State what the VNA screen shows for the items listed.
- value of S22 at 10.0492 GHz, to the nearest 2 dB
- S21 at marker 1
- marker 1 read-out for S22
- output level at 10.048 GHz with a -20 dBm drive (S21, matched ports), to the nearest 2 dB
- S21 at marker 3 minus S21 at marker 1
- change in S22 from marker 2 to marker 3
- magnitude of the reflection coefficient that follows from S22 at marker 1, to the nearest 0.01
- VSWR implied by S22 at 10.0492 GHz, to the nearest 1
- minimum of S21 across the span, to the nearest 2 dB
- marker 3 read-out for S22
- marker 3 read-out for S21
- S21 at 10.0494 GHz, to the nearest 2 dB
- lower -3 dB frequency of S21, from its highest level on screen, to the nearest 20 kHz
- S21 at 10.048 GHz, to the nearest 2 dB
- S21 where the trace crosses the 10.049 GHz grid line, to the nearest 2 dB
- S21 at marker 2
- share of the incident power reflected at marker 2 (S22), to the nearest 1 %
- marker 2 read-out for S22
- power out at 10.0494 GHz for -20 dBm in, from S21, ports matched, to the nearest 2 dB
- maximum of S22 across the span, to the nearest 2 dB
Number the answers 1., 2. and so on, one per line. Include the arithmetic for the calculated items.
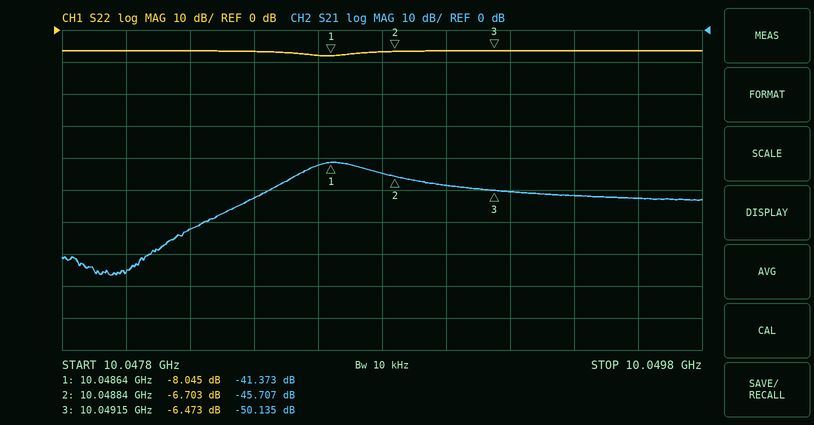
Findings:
1. -6 dB
2. -41.373 dB
3. -8.045 dB
4. -20 dBm + (-76 dB) = -96 dBm
5. -50.135 − (-41.373) = -8.762 dB
6. -6.473 − (-6.703) = 0.230 dB
7. 10^(-8.045/20) ≈ 0.40
8. |Γ| = 10^(-6/20) = 0.5012; VSWR = (1 + 0.5012)/(1 − 0.5012) ≈ 3
9. -76 dB
10. -6.473 dB
11. -50.135 dB
12. -52 dB
13. 10.04856 GHz
14. -76 dB
15. -48 dB
16. -45.707 dB
17. 10^(-6.703/10) ≈ 21 %
18. -6.703 dB
19. -20 dBm + (-52 dB) = -72 dBm
20. -6 dB
